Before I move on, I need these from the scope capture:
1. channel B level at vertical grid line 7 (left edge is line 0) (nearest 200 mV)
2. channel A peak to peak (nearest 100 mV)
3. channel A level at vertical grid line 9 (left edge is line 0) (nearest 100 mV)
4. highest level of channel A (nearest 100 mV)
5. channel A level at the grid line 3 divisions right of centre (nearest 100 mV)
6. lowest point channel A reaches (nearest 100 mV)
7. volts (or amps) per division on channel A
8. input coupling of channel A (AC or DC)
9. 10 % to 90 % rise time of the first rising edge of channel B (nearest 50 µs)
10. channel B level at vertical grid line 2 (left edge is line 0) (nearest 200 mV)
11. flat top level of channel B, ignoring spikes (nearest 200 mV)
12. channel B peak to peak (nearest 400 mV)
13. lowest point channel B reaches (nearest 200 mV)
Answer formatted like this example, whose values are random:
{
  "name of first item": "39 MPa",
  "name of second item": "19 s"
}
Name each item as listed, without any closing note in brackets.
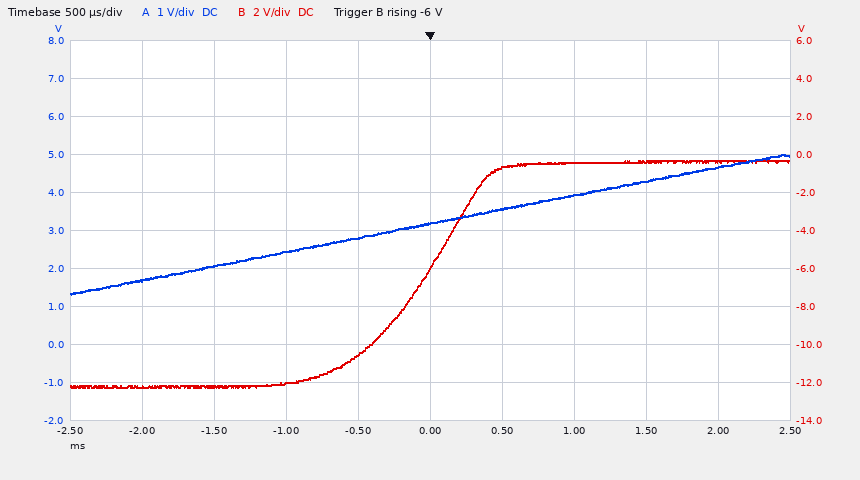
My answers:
{
  "channel B level at vertical grid line 7 (left edge is line 0)": "-400 mV",
  "channel A peak to peak": "3.7 V",
  "channel A level at vertical grid line 9 (left edge is line 0)": "4.7 V",
  "highest level of channel A": "5.0 V",
  "channel A level at the grid line 3 divisions right of centre": "4.3 V",
  "lowest point channel A reaches": "1.3 V",
  "volts (or amps) per division on channel A": "1 V",
  "input coupling of channel A": "DC",
  "10 % to 90 % rise time of the first rising edge of channel B": "950 µs",
  "channel B level at vertical grid line 2 (left edge is line 0)": "-12.2 V",
  "flat top level of channel B, ignoring spikes": "-400 mV",
  "channel B peak to peak": "12.0 V",
  "lowest point channel B reaches": "-12.2 V"
}
